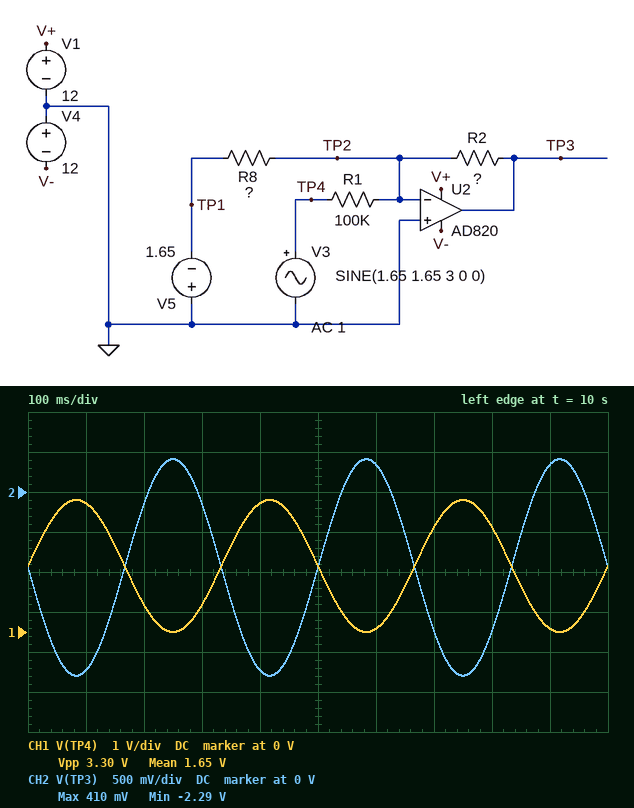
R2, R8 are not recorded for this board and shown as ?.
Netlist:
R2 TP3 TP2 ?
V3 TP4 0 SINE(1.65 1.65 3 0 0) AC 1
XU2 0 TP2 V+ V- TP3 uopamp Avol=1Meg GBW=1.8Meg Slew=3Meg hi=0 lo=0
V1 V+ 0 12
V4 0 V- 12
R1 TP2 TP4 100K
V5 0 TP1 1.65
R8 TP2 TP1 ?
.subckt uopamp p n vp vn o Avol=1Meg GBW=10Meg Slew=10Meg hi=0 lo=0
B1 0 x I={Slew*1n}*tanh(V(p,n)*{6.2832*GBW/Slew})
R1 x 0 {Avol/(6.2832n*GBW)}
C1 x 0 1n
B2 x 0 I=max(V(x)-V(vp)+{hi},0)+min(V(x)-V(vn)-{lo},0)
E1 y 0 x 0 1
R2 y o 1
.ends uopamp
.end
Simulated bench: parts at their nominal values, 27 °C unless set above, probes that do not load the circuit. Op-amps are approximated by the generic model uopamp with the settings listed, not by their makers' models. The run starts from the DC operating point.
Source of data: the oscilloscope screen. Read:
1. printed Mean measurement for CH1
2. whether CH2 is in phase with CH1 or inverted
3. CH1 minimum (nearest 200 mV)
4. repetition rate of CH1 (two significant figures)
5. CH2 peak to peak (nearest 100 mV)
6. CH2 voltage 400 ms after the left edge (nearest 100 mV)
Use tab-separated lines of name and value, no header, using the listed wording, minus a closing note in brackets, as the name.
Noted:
printed Mean measurement for CH1	1.65 V
whether CH2 is in phase with CH1 or inverted	inverted
CH1 minimum	0 V
repetition rate of CH1	3.0 Hz
CH2 peak to peak	2.7 V
CH2 voltage 400 ms after the left edge	-2.2 V
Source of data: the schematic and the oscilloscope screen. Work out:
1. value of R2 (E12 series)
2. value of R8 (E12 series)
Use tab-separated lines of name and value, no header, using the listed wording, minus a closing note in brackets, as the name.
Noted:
value of R2	82 kΩ
value of R8	330 kΩ
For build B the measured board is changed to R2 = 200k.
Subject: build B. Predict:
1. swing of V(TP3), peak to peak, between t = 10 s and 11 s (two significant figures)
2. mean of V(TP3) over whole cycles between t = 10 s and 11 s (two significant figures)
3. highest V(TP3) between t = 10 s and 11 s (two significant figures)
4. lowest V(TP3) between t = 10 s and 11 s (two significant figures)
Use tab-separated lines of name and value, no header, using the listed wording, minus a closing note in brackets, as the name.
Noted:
swing of V(TP3), peak to peak, between t = 10 s and 11 s	6.6 V
mean of V(TP3) over whole cycles between t = 10 s and 11 s	-2.3 V
highest V(TP3) between t = 10 s and 11 s	1.0 V
lowest V(TP3) between t = 10 s and 11 s	-5.6 V
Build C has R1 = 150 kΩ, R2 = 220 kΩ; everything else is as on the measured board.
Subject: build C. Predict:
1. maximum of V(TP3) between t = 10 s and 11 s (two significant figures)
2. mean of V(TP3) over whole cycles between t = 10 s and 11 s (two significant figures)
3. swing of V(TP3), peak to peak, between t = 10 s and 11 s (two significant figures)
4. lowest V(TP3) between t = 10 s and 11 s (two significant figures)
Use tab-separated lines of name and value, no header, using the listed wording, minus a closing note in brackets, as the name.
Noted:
maximum of V(TP3) between t = 10 s and 11 s	1.1 V
mean of V(TP3) over whole cycles between t = 10 s and 11 s	-1.3 V
swing of V(TP3), peak to peak, between t = 10 s and 11 s	4.8 V
lowest V(TP3) between t = 10 s and 11 s	-3.7 V
